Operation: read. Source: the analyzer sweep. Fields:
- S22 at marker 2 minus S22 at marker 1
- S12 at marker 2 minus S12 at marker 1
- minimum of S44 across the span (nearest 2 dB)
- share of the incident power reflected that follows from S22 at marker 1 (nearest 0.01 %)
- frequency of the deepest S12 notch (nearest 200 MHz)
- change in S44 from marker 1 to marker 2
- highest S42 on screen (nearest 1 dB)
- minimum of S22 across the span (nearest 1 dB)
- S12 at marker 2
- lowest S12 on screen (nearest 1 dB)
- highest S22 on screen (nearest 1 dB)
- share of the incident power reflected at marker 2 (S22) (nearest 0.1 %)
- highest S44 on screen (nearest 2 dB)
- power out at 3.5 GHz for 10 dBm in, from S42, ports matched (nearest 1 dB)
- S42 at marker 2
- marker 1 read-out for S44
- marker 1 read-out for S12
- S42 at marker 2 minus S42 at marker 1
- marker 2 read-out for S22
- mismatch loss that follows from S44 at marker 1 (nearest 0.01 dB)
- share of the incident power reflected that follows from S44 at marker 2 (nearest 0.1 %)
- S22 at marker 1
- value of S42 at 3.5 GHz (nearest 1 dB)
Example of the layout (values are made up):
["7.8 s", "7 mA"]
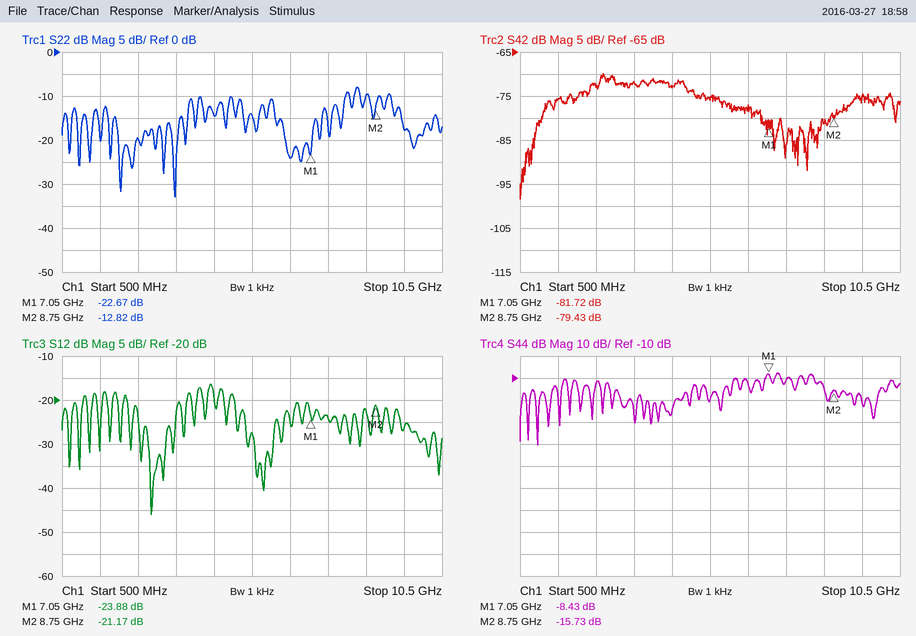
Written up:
["9.85 dB", "2.71 dB", "-40 dB", "0.54 %", "2.8 GHz", "-7.30 dB", "-70 dB", "-33 dB", "-21.17 dB", "-46 dB", "-8 dB", "5.2 %", "-8 dB", "-62 dBm", "-79.43 dB", "-8.43 dB", "-23.88 dB", "2.29 dB", "-12.82 dB", "0.67 dB", "2.7 %", "-22.67 dB", "-72 dB"]
